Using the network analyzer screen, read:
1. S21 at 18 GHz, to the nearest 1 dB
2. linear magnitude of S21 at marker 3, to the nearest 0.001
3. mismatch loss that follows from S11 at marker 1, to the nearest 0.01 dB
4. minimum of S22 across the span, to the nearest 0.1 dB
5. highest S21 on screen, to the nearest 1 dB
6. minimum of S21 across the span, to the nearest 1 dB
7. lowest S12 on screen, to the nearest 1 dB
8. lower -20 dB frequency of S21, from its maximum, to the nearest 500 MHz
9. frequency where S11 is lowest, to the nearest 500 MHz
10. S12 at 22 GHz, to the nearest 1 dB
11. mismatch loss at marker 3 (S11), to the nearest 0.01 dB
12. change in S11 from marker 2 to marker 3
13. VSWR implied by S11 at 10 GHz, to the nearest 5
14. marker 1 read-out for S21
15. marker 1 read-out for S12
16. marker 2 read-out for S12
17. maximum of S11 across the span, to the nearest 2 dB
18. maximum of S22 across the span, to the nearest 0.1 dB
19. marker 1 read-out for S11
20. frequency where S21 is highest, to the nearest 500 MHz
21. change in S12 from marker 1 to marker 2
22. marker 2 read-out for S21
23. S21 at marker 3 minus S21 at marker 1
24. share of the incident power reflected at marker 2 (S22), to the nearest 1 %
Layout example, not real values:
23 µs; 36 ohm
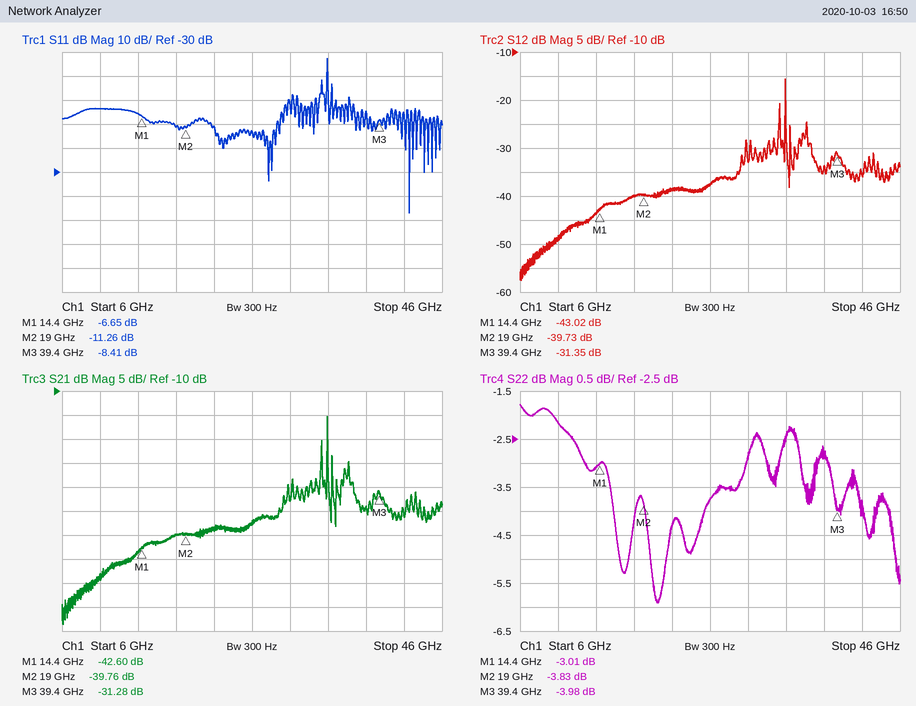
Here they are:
-40 dB; 0.027; 1.06 dB; -5.9 dB; -15 dB; -59 dB; -58 dB; 29.0 GHz; 42.5 GHz; -39 dB; 0.68 dB; 2.85 dB; 5; -42.60 dB; -43.02 dB; -39.73 dB; 18 dB; -1.8 dB; -6.65 dB; 34.0 GHz; 3.29 dB; -39.76 dB; 11.32 dB; 41 %
